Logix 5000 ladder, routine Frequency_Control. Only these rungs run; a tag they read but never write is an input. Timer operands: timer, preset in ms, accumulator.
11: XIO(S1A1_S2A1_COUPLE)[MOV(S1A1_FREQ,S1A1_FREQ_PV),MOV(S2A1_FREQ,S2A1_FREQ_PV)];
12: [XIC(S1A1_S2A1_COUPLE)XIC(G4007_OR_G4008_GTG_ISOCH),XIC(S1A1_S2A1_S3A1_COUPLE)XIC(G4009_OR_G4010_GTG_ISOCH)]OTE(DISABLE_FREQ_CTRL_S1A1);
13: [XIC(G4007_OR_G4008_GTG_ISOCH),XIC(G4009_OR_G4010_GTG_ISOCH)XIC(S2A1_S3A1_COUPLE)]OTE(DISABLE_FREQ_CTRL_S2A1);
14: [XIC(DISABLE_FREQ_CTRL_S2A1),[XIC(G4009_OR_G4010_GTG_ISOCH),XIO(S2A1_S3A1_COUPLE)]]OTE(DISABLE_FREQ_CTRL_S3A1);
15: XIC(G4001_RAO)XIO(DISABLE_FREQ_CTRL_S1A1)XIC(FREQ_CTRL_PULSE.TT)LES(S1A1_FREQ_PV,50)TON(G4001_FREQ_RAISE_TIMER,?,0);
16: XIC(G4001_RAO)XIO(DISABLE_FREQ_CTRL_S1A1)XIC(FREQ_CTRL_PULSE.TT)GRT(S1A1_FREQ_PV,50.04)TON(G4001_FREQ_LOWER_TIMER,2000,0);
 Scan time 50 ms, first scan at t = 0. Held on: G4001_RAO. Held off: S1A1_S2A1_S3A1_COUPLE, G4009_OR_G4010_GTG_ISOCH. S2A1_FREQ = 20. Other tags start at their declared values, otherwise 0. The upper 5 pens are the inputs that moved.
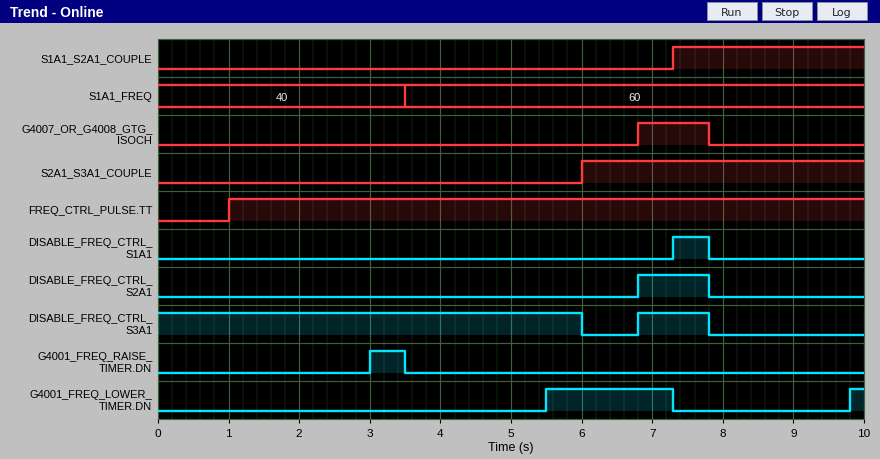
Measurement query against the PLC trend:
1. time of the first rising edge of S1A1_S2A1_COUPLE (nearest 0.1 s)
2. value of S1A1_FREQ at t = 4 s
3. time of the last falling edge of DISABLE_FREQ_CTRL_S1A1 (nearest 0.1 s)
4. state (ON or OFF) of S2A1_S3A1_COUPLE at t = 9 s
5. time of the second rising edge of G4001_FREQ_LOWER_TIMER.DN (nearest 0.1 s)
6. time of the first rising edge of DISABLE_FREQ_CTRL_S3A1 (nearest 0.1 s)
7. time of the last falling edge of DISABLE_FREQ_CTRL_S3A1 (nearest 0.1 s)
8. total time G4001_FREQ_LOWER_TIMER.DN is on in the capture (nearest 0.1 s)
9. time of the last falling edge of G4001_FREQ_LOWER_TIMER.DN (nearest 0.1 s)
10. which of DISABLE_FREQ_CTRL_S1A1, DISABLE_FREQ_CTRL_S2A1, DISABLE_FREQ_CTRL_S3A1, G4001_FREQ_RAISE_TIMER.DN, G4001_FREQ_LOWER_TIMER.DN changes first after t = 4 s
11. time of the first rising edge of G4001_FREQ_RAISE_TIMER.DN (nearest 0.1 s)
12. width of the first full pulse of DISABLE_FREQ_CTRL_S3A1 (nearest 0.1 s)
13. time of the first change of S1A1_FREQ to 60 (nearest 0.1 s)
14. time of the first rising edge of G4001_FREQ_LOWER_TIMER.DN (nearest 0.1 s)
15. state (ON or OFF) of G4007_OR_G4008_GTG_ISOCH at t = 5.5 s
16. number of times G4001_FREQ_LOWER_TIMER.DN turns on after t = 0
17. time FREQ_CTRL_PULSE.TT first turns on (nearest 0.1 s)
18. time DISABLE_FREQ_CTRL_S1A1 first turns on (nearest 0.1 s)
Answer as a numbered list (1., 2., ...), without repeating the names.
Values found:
1. 7.3 s
2. 60
3. 7.8 s
4. ON
5. 9.8 s
6. 6.8 s
7. 7.8 s
8. 2.0 s
9. 7.3 s
10. G4001_FREQ_LOWER_TIMER.DN
11. 3.0 s
12. 1.0 s
13. 3.5 s
14. 5.5 s
15. OFF
16. 2
17. 1.0 s
18. 7.3 s
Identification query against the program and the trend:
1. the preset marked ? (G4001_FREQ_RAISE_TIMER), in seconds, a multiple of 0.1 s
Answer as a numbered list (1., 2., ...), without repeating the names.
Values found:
1. 2.0 s
